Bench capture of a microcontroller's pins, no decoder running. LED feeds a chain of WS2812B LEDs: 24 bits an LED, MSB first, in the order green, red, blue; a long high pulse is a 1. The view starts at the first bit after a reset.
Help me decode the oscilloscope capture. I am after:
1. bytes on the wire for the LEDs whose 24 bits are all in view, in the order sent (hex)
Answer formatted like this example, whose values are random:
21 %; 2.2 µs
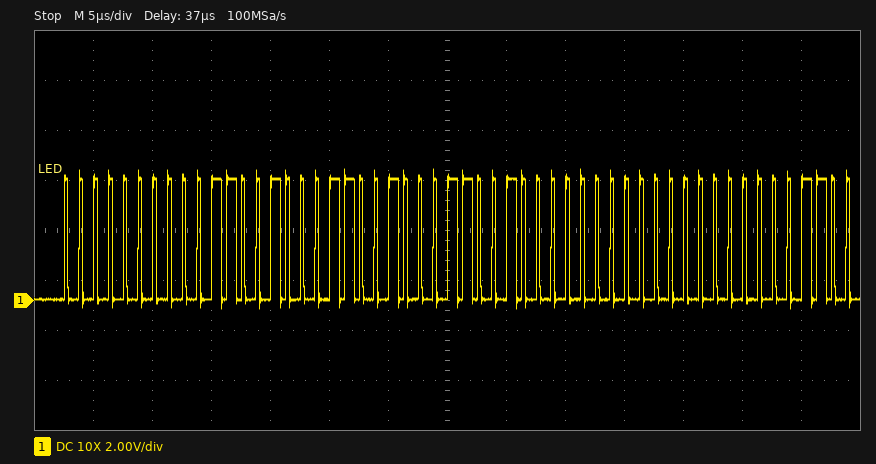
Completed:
00 32 32 32 00 00
